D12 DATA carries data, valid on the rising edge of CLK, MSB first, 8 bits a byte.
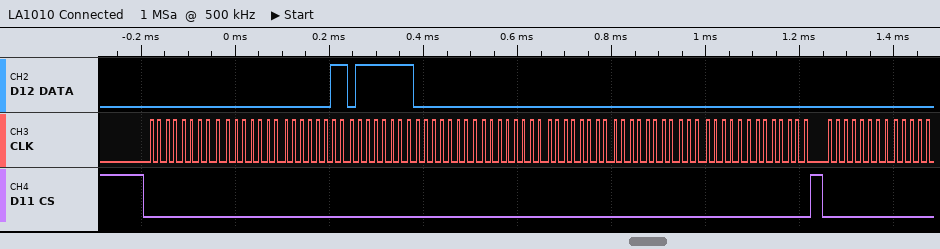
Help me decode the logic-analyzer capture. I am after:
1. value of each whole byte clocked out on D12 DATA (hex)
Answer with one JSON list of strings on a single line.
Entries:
["00 00 03 7F 00 00 00 00 00 00 00"]
